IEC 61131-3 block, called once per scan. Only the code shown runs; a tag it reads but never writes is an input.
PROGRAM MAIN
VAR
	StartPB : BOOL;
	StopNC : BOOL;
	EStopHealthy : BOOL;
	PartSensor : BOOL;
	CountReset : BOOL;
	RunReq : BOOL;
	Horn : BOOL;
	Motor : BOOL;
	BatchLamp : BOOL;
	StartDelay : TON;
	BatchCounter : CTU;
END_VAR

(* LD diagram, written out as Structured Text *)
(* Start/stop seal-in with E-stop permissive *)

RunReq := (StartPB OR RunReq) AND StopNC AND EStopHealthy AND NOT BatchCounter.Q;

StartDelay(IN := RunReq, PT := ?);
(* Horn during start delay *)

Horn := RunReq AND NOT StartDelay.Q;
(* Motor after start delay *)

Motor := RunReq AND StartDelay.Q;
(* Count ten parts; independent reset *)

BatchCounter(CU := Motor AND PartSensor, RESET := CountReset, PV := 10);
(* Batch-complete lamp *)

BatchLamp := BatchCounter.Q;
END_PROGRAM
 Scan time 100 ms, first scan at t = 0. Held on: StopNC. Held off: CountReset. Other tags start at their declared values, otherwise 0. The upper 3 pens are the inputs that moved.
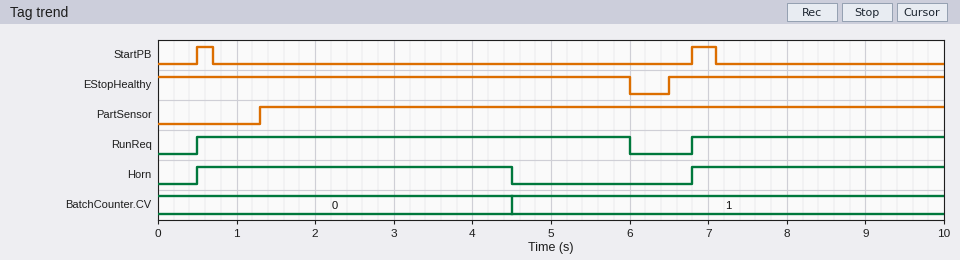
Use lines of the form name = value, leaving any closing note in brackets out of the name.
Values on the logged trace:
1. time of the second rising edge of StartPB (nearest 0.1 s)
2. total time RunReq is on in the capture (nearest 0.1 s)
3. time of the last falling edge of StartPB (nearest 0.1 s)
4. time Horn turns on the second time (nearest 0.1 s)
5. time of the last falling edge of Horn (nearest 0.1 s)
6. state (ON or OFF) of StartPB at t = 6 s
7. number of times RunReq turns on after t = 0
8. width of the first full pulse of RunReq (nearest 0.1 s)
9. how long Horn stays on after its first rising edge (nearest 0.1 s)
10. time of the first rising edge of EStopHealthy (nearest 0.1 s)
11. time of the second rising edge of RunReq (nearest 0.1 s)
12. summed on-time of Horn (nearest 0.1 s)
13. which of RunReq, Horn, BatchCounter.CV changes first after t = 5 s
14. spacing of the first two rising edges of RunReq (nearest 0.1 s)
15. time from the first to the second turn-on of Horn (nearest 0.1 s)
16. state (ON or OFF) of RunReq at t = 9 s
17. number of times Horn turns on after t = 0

time of the second rising edge of StartPB = 6.8 s
total time RunReq is on in the capture = 8.7 s
time of the last falling edge of StartPB = 7.1 s
time Horn turns on the second time = 6.8 s
time of the last falling edge of Horn = 4.5 s
state (ON or OFF) of StartPB at t = 6 s = OFF
number of times RunReq turns on after t = 0 = 2
width of the first full pulse of RunReq = 5.5 s
how long Horn stays on after its first rising edge = 4.0 s
time of the first rising edge of EStopHealthy = 6.5 s
time of the second rising edge of RunReq = 6.8 s
summed on-time of Horn = 7.2 s
which of RunReq, Horn, BatchCounter.CV changes first after t = 5 s = RunReq
spacing of the first two rising edges of RunReq = 6.3 s
time from the first to the second turn-on of Horn = 6.3 s
state (ON or OFF) of RunReq at t = 9 s = ON
number of times Horn turns on after t = 0 = 2
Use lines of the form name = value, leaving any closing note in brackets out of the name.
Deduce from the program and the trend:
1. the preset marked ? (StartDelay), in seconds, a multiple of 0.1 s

the preset marked ? (StartDelay), in seconds, a multiple of 0.1 s = 4.0 s
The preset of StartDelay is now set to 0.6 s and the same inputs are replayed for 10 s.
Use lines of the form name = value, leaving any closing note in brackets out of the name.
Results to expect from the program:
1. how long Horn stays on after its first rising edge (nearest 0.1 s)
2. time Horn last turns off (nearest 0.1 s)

how long Horn stays on after its first rising edge = 0.6 s
time Horn last turns off = 7.4 s
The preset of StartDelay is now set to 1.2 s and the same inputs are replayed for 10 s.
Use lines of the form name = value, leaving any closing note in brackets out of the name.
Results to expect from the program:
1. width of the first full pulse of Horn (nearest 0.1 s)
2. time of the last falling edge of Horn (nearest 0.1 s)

width of the first full pulse of Horn = 1.2 s
time of the last falling edge of Horn = 8.0 s
